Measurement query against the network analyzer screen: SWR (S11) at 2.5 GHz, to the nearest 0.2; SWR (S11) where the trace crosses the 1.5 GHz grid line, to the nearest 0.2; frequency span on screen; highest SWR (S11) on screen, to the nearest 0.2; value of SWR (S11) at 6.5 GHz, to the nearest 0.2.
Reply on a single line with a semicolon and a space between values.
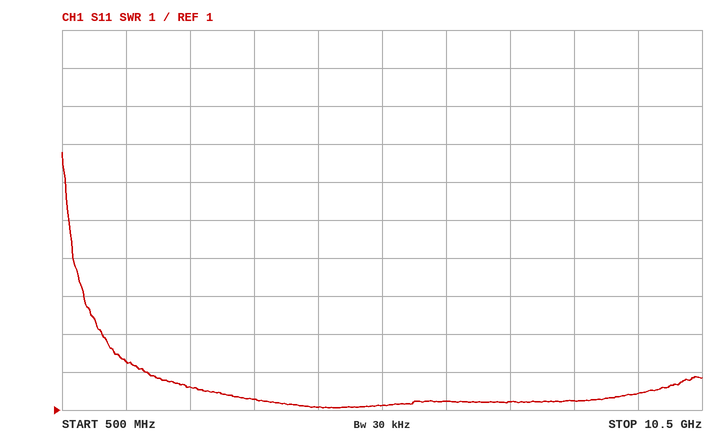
1.6; 2.2; 10 GHz; 7.8; 1.2
